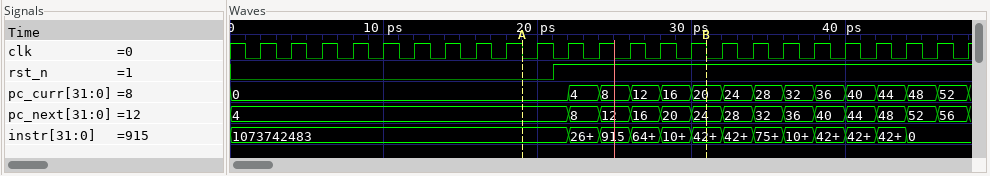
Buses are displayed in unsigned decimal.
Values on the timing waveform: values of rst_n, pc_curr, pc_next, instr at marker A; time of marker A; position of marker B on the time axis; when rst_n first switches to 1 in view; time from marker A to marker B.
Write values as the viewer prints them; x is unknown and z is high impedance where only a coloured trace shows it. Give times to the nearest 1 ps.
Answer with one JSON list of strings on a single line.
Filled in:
["rst_n=0, pc_curr=0, pc_next=4, instr=1073742483", "19 ps", "31 ps", "21 ps", "12 ps"]
